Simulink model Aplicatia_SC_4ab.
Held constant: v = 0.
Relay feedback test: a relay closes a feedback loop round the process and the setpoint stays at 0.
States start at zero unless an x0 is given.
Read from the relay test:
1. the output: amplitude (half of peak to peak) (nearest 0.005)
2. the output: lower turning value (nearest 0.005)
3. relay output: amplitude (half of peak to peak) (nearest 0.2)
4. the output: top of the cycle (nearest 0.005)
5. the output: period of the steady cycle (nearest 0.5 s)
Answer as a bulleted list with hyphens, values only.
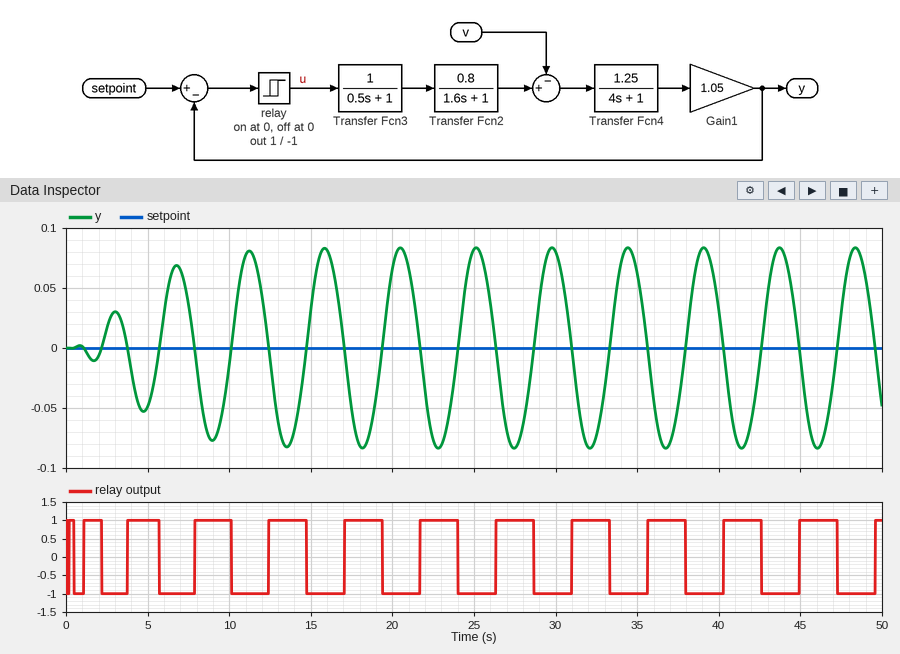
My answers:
- 0.085
- -0.085
- 1.0
- 0.085
- 4.5 s
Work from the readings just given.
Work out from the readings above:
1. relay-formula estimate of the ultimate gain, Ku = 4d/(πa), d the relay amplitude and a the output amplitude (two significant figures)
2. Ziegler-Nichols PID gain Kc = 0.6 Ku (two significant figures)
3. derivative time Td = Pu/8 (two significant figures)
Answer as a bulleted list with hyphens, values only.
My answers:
- 15
- 9.0
- 0.56 s
